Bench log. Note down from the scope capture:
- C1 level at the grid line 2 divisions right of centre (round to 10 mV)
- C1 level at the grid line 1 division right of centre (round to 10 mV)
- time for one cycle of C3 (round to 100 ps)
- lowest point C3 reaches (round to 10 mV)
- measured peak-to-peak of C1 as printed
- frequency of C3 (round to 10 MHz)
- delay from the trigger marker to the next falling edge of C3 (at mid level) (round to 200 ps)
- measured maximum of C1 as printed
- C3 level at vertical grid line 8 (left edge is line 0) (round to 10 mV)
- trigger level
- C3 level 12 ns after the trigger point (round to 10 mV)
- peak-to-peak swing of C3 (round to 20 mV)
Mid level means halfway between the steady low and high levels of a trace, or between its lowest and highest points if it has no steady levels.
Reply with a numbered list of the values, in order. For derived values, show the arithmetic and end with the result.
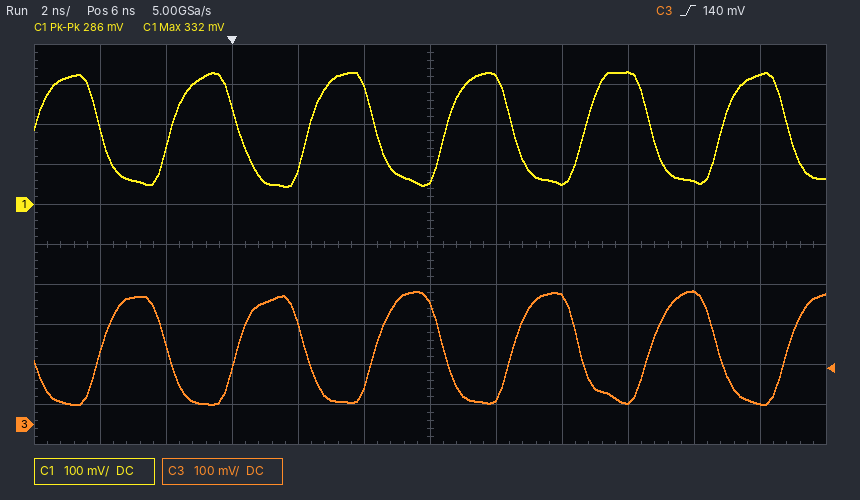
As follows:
1. 50 mV
2. 320 mV
3. 4.2 ns
4. 50 mV
5. 286 mV
6. 1 / 4.2 ns ≈ 238 MHz, so 240 MHz to the nearest 10 MHz
7. 2.2 ns
8. 332 mV
9. 320 mV
10. 140 mV
11. 60 mV
12. 280 mV
